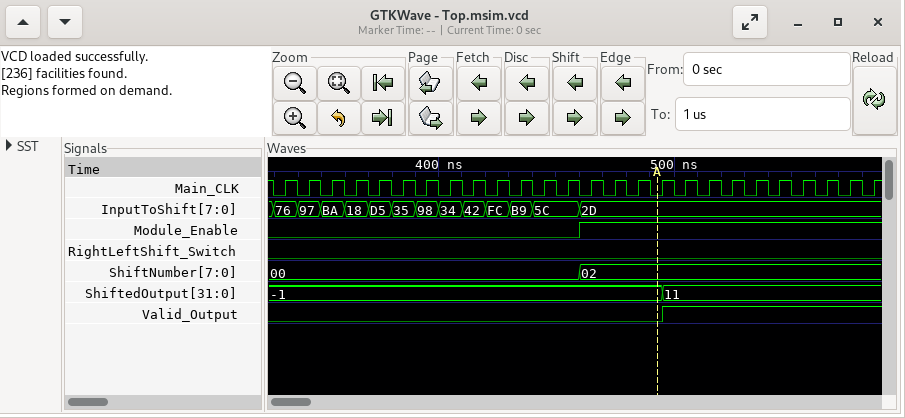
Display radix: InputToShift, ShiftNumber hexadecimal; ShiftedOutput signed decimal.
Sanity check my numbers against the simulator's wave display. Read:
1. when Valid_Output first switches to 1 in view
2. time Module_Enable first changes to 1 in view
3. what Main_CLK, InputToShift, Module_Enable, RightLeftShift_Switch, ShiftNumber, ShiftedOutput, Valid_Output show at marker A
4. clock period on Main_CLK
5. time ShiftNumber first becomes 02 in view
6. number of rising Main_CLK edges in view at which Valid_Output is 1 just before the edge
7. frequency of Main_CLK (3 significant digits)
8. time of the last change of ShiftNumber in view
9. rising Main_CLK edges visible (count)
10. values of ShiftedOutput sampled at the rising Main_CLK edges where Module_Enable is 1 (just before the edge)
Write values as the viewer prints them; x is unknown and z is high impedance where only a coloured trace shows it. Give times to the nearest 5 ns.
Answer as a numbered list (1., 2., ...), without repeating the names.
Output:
1. 495 ns
2. 460 ns
3. Main_CLK=0, InputToShift=2D, Module_Enable=1, RightLeftShift_Switch=0, ShiftNumber=02, ShiftedOutput=-1, Valid_Output=0
4. 10 ns
5. 460 ns
6. 9
7. 100 MHz
8. 460 ns
9. 26
10. -1, -1, -1, -1, 11, 11, 11, 11, 11, 11, 11, 11, 11
